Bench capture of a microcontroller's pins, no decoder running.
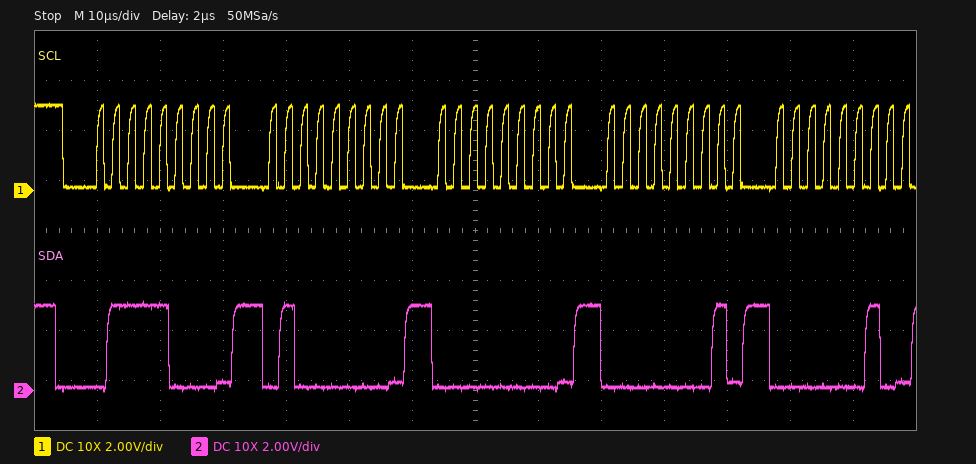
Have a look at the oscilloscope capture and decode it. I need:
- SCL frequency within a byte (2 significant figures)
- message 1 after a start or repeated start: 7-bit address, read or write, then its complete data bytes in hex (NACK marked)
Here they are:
400 kHz
0x3C write: 40 00 01 02
